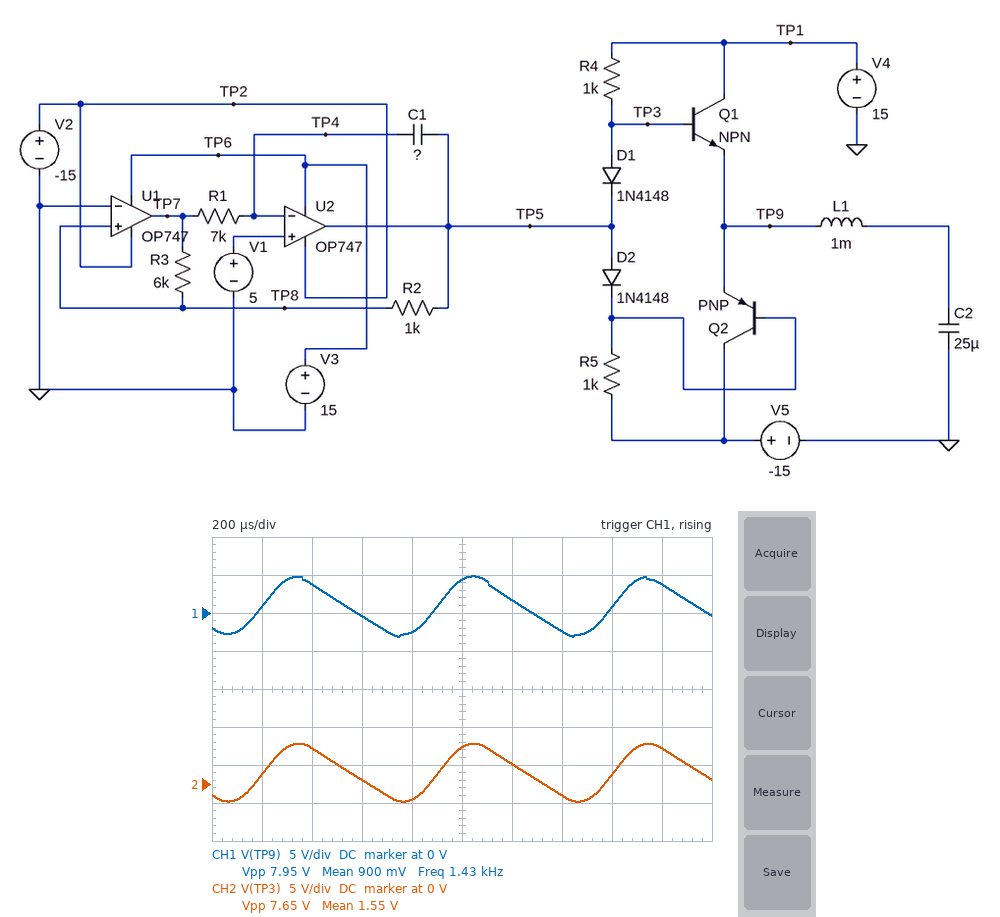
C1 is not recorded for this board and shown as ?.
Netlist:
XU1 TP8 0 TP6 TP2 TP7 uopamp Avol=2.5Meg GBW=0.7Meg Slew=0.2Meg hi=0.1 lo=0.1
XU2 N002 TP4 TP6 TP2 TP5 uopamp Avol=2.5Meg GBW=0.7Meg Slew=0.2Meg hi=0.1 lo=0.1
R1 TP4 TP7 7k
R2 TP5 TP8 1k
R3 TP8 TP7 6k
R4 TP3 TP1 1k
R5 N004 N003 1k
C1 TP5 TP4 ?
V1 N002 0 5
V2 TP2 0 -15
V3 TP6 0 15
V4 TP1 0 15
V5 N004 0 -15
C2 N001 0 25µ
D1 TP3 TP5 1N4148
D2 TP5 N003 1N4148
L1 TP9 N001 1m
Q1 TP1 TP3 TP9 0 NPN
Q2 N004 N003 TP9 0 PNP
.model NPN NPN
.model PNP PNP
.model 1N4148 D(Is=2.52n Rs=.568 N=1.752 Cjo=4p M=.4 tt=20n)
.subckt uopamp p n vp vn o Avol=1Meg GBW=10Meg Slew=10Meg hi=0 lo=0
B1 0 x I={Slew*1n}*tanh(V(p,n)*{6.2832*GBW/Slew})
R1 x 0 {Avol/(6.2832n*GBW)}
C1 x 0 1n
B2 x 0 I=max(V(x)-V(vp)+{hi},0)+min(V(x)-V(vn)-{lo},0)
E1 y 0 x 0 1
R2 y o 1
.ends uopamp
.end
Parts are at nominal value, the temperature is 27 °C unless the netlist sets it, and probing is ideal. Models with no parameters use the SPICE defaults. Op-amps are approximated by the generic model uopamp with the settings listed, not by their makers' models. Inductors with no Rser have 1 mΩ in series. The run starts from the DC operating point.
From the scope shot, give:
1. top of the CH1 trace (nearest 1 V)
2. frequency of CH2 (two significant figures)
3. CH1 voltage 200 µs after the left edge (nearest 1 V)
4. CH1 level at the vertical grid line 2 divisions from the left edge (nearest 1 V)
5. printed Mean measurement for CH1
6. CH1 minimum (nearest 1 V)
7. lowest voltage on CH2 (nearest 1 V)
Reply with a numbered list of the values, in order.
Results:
1. 5 V
2. 1.4 kHz
3. 1 V
4. 4 V
5. 900 mV
6. -3 V
7. -2 V
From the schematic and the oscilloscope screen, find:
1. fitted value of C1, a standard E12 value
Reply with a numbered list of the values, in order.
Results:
1. 68 nF
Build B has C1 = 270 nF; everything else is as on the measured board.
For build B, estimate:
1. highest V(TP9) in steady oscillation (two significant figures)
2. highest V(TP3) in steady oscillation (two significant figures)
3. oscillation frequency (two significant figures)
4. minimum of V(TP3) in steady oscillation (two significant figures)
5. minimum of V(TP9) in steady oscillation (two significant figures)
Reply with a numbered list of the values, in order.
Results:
1. 2.8 V
2. 3.7 V
3. 570 Hz
4. -1.9 V
5. -2.8 V
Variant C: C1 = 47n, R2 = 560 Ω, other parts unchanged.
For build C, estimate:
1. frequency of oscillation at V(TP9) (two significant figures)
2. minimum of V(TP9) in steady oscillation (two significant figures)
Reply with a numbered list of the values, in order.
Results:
1. 2.1 kHz
2. -2.3 V
